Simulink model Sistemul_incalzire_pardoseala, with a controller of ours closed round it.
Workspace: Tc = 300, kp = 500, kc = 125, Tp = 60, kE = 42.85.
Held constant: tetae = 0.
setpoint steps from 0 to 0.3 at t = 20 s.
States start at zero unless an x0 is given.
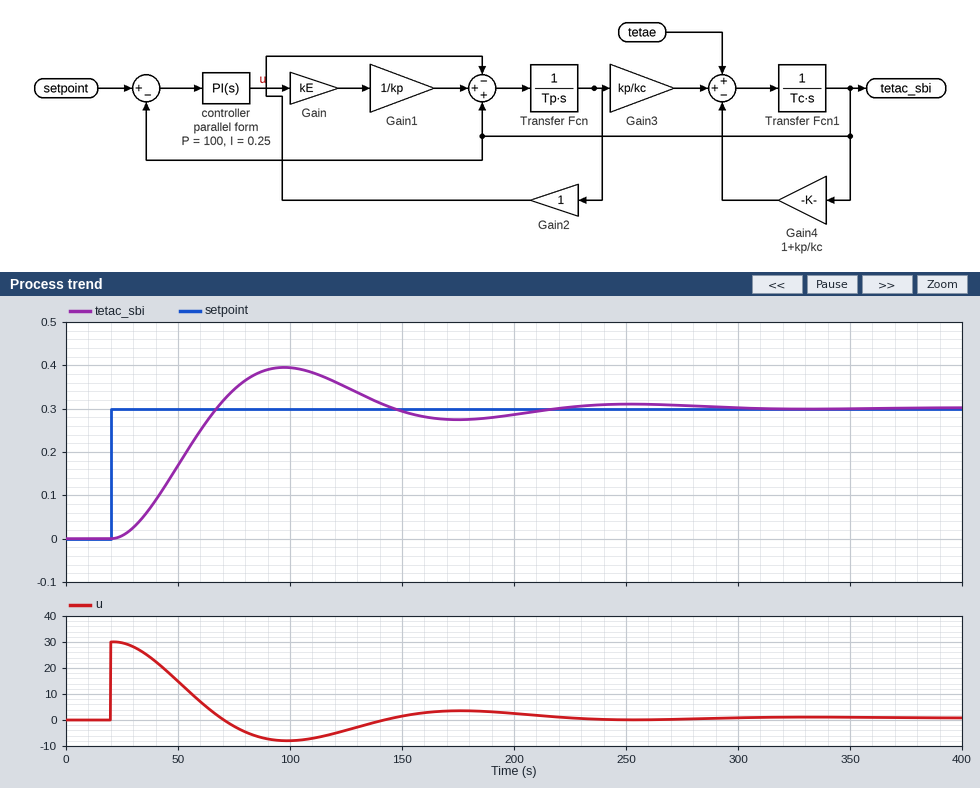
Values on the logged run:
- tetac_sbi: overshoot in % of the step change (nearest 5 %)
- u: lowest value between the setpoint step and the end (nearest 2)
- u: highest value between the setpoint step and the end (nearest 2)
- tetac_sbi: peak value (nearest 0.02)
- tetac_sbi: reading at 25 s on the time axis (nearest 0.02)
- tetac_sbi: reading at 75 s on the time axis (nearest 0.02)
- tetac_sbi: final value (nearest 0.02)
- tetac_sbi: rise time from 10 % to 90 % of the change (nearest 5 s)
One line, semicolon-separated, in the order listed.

30 %; -8; 30; 0.40; 0.00; 0.34; 0.30; 30 s
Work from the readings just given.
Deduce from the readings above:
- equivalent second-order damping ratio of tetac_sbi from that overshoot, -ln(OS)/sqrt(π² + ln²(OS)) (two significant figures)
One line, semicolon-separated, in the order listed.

0.36
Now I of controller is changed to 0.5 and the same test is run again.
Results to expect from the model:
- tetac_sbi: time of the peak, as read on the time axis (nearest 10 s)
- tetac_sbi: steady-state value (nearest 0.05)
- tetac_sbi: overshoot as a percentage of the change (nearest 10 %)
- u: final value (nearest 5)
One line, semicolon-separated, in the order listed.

100 s; 0.30; 40 %; 0
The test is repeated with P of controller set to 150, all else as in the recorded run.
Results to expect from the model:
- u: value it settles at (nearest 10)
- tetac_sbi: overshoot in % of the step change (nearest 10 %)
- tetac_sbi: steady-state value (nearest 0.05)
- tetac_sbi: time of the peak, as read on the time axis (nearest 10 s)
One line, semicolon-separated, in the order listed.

0; 40 %; 0.30; 80 s
